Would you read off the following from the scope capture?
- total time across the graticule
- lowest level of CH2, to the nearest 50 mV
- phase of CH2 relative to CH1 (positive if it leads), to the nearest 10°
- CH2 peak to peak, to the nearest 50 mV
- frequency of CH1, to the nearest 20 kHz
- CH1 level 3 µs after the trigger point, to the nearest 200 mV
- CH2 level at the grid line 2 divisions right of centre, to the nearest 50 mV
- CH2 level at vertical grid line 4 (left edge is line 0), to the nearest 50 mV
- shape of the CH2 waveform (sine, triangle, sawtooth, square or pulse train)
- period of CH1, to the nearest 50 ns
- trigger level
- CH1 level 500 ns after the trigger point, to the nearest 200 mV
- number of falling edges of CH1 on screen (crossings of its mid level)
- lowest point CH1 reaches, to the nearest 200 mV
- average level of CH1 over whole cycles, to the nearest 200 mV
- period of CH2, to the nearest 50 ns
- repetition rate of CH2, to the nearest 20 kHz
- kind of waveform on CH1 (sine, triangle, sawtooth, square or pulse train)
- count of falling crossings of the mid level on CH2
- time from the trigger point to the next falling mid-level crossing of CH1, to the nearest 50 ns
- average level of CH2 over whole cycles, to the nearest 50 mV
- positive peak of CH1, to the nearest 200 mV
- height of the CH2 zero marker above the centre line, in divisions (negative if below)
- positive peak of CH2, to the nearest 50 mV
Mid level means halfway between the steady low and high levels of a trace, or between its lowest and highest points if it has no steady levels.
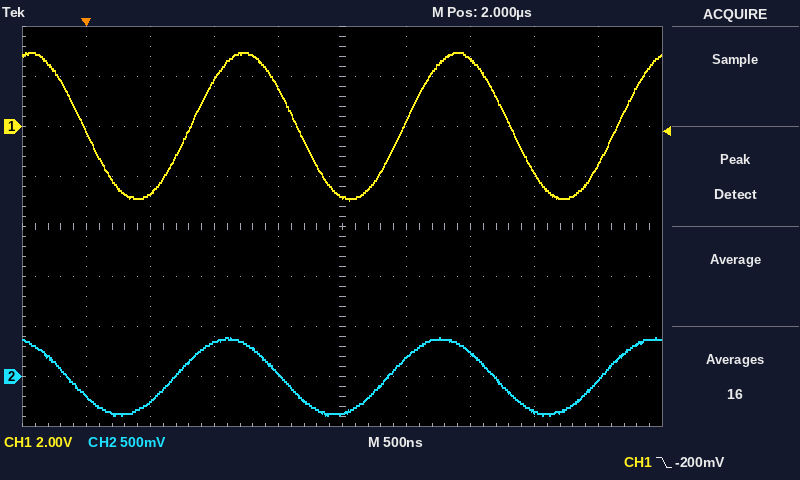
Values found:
5 µs
-400 mV
+30°
800 mV
600 kHz
2.6 V
250 mV
50 mV
sine
1.65 µs
-200 mV
-2.6 V
3
-3.0 V
0.0 V
1.65 µs
600 kHz
sine
3
1.65 µs
0 mV
3.0 V
-3.0 div
400 mV
